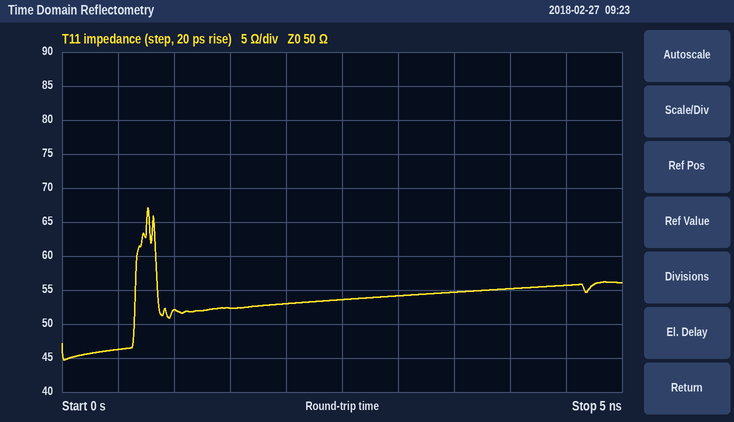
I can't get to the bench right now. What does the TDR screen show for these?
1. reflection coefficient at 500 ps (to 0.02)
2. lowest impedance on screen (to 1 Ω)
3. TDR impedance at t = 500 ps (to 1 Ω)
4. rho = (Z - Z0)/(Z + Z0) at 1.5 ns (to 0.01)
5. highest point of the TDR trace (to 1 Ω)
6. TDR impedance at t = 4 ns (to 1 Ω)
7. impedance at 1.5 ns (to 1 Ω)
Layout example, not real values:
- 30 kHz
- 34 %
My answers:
- -0.04
- 45 Ω
- 46 Ω
- +0.02
- 67 Ω
- 55 Ω
- 52 Ω
